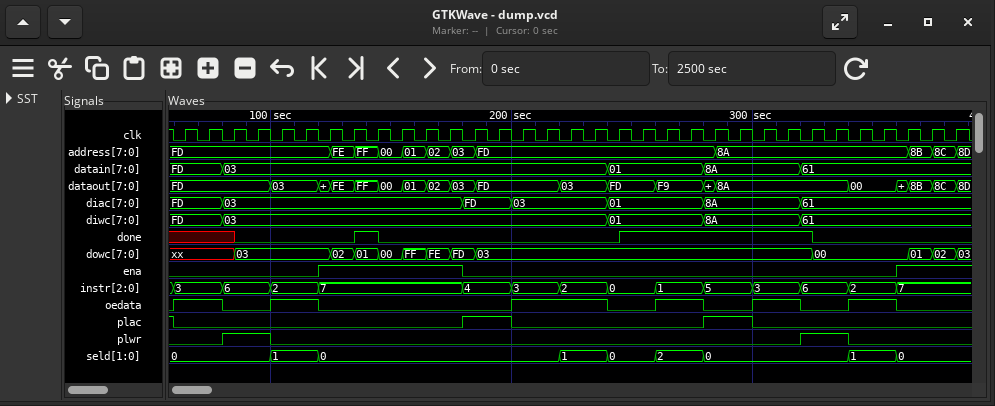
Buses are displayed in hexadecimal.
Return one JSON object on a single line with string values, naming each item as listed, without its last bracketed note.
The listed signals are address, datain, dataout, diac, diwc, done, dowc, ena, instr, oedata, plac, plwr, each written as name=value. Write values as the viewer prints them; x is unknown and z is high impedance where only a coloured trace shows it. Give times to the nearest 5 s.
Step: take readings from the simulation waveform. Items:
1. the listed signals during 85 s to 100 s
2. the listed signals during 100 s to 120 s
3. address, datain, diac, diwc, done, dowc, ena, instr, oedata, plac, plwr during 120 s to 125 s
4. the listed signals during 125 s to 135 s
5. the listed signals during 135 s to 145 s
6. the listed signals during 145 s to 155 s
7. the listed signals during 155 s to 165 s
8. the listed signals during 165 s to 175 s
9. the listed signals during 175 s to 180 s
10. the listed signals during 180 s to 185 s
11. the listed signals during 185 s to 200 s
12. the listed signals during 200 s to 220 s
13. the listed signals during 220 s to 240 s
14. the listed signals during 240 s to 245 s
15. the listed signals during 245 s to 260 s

{"the listed signals during 85 s to 100 s": "address=FD, datain=03, dataout=FD, diac=03, diwc=03, done=0, dowc=03, ena=0, instr=6, oedata=0, plac=0, plwr=1", "the listed signals during 100 s to 120 s": "address=FD, datain=03, dataout=03, diac=03, diwc=03, done=0, dowc=03, ena=0, instr=2, oedata=1, plac=0, plwr=0", "address, datain, diac, diwc, done, dowc, ena, instr, oedata, plac, plwr during 120 s to 125 s": "address=FD, datain=03, diac=03, diwc=03, done=0, dowc=03, ena=1, instr=7, oedata=0, plac=0, plwr=0", "the listed signals during 125 s to 135 s": "address=FE, datain=03, dataout=FE, diac=03, diwc=03, done=0, dowc=02, ena=1, instr=7, oedata=0, plac=0, plwr=0", "the listed signals during 135 s to 145 s": "address=FF, datain=03, dataout=FF, diac=03, diwc=03, done=1, dowc=01, ena=1, instr=7, oedata=0, plac=0, plwr=0", "the listed signals during 145 s to 155 s": "address=00, datain=03, dataout=00, diac=03, diwc=03, done=0, dowc=00, ena=1, instr=7, oedata=0, plac=0, plwr=0", "the listed signals during 155 s to 165 s": "address=01, datain=03, dataout=01, diac=03, diwc=03, done=0, dowc=FF, ena=1, instr=7, oedata=0, plac=0, plwr=0", "the listed signals during 165 s to 175 s": "address=02, datain=03, dataout=02, diac=03, diwc=03, done=0, dowc=FE, ena=1, instr=7, oedata=0, plac=0, plwr=0", "the listed signals during 175 s to 180 s": "address=03, datain=03, dataout=03, diac=03, diwc=03, done=0, dowc=FD, ena=1, instr=7, oedata=0, plac=0, plwr=0", "the listed signals during 180 s to 185 s": "address=03, datain=03, dataout=03, diac=FD, diwc=03, done=0, dowc=FD, ena=0, instr=4, oedata=0, plac=1, plwr=0", "the listed signals during 185 s to 200 s": "address=FD, datain=03, dataout=FD, diac=FD, diwc=03, done=0, dowc=03, ena=0, instr=4, oedata=0, plac=1, plwr=0", "the listed signals during 200 s to 220 s": "address=FD, datain=03, dataout=FD, diac=03, diwc=03, done=0, dowc=03, ena=0, instr=3, oedata=1, plac=0, plwr=0", "the listed signals during 220 s to 240 s": "address=FD, datain=03, dataout=03, diac=03, diwc=03, done=0, dowc=03, ena=0, instr=2, oedata=1, plac=0, plwr=0", "the listed signals during 240 s to 245 s": "address=FD, datain=01, dataout=FD, diac=01, diwc=01, done=0, dowc=03, ena=0, instr=0, oedata=0, plac=0, plwr=0", "the listed signals during 245 s to 260 s": "address=FD, datain=01, dataout=FD, diac=01, diwc=01, done=1, dowc=03, ena=0, instr=0, oedata=0, plac=0, plwr=0"}
